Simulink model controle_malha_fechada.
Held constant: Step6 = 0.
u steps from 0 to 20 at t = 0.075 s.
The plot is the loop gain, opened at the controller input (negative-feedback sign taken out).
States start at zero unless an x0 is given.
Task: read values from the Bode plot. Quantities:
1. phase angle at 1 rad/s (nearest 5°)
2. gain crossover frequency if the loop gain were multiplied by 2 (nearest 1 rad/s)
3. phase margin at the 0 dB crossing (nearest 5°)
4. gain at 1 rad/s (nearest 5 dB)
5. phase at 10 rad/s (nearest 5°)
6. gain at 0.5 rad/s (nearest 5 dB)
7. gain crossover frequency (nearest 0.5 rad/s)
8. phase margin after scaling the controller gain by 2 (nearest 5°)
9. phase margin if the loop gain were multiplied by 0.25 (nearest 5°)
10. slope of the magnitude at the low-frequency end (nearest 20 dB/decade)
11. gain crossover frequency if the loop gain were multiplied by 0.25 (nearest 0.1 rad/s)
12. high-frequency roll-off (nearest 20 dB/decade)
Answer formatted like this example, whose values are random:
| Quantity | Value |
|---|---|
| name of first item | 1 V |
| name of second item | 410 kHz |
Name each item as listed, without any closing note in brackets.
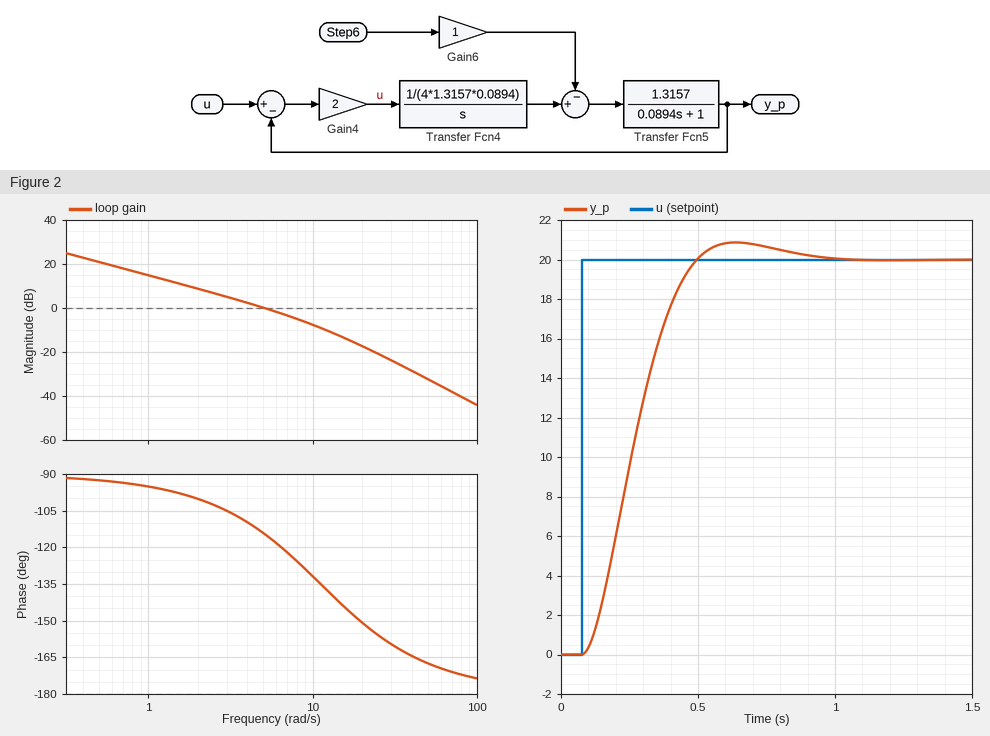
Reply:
| Quantity | Value |
|---|---|
| phase angle at 1 rad/s | -95° |
| gain crossover frequency if the loop gain were multiplied by 2 | 9 rad/s |
| phase margin at the 0 dB crossing | 65° |
| gain at 1 rad/s | 15 dB |
| phase at 10 rad/s | -130° |
| gain at 0.5 rad/s | 20 dB |
| gain crossover frequency | 5.0 rad/s |
| phase margin after scaling the controller gain by 2 | 50° |
| phase margin if the loop gain were multiplied by 0.25 | 85° |
| slope of the magnitude at the low-frequency end | -20 dB/decade |
| gain crossover frequency if the loop gain were multiplied by 0.25 | 1.4 rad/s |
| high-frequency roll-off | -40 dB/decade |
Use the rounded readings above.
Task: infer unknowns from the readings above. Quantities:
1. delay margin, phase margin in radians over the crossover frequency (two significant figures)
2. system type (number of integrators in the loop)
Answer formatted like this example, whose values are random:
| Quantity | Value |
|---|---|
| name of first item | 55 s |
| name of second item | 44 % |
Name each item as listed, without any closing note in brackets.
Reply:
| Quantity | Value |
|---|---|
| delay margin, phase margin in radians over the crossover frequency | 0.23 s |
| system type | 1 |
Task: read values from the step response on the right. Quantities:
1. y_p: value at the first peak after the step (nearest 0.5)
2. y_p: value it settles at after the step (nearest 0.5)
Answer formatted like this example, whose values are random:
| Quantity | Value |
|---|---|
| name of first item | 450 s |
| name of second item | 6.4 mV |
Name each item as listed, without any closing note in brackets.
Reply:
| Quantity | Value |
|---|---|
| y_p: value at the first peak after the step | 21.0 |
| y_p: value it settles at after the step | 20.0 |
